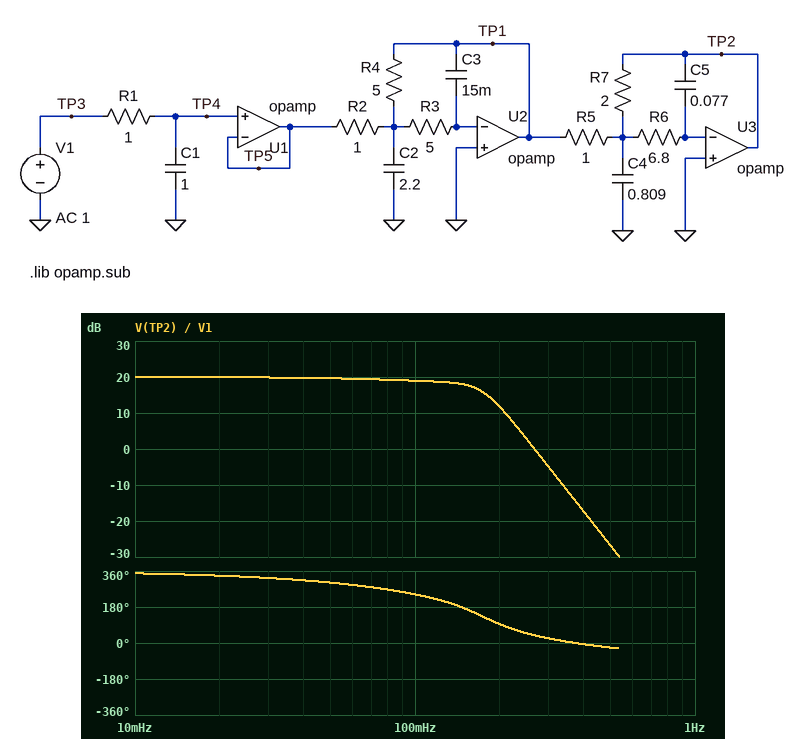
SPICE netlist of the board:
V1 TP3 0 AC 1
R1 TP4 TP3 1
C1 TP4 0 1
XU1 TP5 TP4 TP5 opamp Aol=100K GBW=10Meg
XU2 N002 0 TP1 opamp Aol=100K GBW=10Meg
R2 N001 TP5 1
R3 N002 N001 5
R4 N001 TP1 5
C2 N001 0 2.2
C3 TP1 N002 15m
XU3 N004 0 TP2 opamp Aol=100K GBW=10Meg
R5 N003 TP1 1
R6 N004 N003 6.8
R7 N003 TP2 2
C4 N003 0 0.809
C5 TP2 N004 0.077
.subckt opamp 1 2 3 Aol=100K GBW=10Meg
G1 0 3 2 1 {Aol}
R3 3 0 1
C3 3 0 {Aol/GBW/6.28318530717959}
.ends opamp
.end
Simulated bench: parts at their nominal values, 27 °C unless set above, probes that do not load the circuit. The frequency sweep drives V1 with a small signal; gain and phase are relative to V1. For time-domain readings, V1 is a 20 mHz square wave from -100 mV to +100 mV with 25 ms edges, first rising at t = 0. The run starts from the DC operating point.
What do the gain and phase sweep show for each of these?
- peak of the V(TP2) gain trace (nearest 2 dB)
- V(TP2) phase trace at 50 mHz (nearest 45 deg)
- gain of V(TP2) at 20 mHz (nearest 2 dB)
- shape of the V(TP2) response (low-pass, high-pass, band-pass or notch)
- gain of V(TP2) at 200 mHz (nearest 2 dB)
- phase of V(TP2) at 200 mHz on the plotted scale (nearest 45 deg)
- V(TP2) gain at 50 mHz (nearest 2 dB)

20 dB
315 deg
20 dB
low-pass
12 dB
90 deg
20 dB
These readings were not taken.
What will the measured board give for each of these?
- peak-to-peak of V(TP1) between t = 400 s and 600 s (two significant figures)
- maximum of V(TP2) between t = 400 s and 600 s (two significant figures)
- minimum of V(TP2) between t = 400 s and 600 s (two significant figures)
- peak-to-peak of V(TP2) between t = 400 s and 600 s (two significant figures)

1.4 V
1.1 V
-1.1 V
2.3 V
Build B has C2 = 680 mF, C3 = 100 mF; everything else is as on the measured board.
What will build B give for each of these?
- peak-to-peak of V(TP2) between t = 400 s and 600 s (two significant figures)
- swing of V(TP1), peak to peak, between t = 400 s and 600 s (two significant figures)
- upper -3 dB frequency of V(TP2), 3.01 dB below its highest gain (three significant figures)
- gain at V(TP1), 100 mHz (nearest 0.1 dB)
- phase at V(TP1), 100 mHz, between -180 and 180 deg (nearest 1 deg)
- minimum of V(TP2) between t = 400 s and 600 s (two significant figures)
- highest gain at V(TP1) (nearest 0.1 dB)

2.0 V
1.0 V
43.8 mHz
5.6 dB
66 deg
-1.0 V
14.0 dB
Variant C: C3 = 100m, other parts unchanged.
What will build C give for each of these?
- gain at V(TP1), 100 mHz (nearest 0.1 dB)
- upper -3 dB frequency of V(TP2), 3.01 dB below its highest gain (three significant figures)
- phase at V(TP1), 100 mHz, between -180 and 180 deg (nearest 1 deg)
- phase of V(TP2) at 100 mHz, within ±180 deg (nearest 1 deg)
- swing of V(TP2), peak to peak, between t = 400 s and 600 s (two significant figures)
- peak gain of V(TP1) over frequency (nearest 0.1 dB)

4.6 dB
54.1 mHz
30 deg
151 deg
2.1 V
14.0 dB
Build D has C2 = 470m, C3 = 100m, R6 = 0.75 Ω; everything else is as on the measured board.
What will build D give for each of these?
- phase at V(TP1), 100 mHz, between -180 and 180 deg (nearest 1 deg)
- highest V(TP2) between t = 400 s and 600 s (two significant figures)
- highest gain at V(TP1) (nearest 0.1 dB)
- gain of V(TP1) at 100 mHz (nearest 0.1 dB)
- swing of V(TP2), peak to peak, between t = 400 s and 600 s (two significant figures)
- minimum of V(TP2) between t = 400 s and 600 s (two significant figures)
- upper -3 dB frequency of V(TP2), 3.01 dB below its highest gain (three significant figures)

72 deg
1.0 V
14.0 dB
5.4 dB
2.0 V
-1.0 V
46.5 mHz
